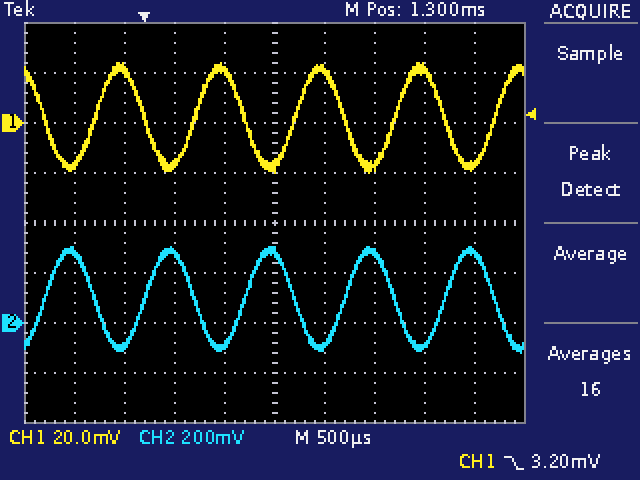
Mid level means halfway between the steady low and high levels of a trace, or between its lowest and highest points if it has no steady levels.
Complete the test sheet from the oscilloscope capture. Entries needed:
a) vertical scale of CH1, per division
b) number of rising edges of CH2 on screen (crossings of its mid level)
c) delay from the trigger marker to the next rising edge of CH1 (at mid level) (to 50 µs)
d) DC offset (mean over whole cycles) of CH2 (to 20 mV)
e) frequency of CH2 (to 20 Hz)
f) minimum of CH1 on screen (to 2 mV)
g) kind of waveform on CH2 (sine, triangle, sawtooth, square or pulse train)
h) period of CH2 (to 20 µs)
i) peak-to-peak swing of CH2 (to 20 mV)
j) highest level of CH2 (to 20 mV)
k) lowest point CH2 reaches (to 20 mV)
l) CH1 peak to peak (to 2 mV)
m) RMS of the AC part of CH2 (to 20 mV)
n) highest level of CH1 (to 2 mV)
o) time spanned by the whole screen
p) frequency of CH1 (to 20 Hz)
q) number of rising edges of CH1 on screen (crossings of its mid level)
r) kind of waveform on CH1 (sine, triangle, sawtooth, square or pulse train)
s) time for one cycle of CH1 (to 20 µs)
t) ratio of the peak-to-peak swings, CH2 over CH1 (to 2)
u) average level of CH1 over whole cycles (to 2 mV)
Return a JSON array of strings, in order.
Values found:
["20 mV", "5", "500 µs", "100 mV", "1.00 kHz", "-20 mV", "sine", "1.00 ms", "420 mV", "300 mV", "-120 mV", "44 mV", "140 mV", "24 mV", "5 ms", "1.00 kHz", "5", "sine", "1.00 ms", "10", "2 mV"]
